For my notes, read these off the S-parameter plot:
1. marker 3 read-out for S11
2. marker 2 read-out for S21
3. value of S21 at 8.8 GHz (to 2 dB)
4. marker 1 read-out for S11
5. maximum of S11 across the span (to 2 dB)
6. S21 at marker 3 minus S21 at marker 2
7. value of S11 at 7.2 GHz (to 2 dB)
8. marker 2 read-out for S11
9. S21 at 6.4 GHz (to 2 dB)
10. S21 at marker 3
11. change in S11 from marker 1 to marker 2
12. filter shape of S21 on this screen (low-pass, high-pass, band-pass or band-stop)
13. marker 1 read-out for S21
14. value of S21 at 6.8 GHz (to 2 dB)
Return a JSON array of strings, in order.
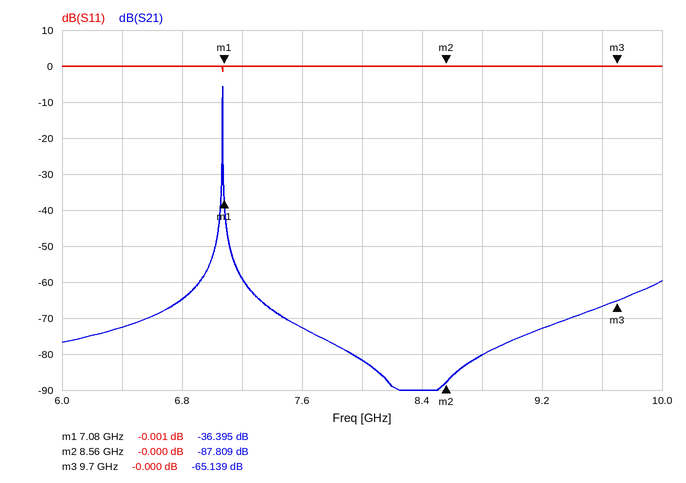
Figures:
["-0.000 dB", "-87.809 dB", "-80 dB", "-0.001 dB", "0 dB", "22.670 dB", "0 dB", "-0.000 dB", "-72 dB", "-65.139 dB", "0.001 dB", "band-pass", "-36.395 dB", "-64 dB"]
